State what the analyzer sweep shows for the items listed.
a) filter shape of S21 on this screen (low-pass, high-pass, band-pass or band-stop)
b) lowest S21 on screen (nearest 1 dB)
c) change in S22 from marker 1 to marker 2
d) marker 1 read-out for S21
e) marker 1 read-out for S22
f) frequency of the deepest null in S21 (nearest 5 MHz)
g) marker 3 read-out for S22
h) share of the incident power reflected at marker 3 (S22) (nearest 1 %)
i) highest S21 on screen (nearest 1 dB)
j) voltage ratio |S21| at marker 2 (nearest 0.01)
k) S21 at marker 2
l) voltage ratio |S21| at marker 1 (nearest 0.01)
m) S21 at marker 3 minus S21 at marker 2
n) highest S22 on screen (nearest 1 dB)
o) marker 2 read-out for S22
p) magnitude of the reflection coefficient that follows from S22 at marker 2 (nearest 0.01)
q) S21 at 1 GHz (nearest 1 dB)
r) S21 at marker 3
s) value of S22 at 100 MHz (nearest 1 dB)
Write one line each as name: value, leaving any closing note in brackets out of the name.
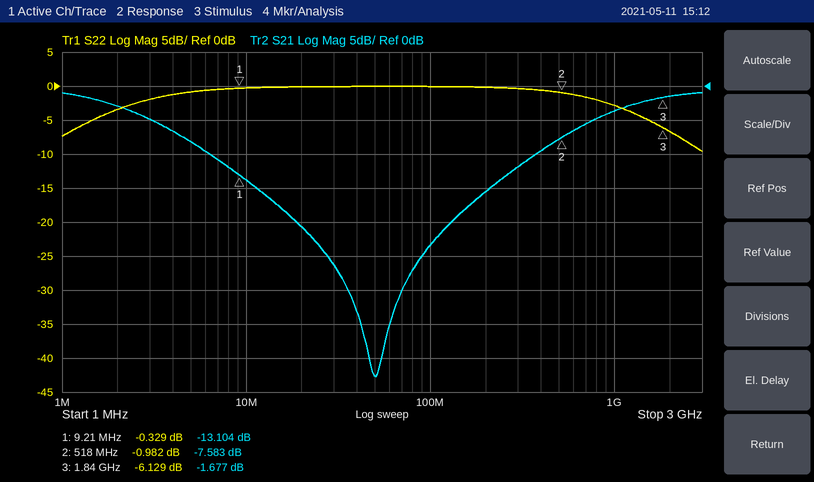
filter shape of S21 on this screen: band-stop
lowest S21 on screen: -43 dB
change in S22 from marker 1 to marker 2: -0.653 dB
marker 1 read-out for S21: -13.104 dB
marker 1 read-out for S22: -0.329 dB
frequency of the deepest null in S21: 50 MHz
marker 3 read-out for S22: -6.129 dB
share of the incident power reflected at marker 3 (S22): 24 %
highest S21 on screen: -1 dB
voltage ratio |S21| at marker 2: 0.42
S21 at marker 2: -7.583 dB
voltage ratio |S21| at marker 1: 0.22
S21 at marker 3 minus S21 at marker 2: 5.906 dB
highest S22 on screen: 0 dB
marker 2 read-out for S22: -0.982 dB
magnitude of the reflection coefficient that follows from S22 at marker 2: 0.89
S21 at 1 GHz: -4 dB
S21 at marker 3: -1.677 dB
value of S22 at 100 MHz: 0 dB
